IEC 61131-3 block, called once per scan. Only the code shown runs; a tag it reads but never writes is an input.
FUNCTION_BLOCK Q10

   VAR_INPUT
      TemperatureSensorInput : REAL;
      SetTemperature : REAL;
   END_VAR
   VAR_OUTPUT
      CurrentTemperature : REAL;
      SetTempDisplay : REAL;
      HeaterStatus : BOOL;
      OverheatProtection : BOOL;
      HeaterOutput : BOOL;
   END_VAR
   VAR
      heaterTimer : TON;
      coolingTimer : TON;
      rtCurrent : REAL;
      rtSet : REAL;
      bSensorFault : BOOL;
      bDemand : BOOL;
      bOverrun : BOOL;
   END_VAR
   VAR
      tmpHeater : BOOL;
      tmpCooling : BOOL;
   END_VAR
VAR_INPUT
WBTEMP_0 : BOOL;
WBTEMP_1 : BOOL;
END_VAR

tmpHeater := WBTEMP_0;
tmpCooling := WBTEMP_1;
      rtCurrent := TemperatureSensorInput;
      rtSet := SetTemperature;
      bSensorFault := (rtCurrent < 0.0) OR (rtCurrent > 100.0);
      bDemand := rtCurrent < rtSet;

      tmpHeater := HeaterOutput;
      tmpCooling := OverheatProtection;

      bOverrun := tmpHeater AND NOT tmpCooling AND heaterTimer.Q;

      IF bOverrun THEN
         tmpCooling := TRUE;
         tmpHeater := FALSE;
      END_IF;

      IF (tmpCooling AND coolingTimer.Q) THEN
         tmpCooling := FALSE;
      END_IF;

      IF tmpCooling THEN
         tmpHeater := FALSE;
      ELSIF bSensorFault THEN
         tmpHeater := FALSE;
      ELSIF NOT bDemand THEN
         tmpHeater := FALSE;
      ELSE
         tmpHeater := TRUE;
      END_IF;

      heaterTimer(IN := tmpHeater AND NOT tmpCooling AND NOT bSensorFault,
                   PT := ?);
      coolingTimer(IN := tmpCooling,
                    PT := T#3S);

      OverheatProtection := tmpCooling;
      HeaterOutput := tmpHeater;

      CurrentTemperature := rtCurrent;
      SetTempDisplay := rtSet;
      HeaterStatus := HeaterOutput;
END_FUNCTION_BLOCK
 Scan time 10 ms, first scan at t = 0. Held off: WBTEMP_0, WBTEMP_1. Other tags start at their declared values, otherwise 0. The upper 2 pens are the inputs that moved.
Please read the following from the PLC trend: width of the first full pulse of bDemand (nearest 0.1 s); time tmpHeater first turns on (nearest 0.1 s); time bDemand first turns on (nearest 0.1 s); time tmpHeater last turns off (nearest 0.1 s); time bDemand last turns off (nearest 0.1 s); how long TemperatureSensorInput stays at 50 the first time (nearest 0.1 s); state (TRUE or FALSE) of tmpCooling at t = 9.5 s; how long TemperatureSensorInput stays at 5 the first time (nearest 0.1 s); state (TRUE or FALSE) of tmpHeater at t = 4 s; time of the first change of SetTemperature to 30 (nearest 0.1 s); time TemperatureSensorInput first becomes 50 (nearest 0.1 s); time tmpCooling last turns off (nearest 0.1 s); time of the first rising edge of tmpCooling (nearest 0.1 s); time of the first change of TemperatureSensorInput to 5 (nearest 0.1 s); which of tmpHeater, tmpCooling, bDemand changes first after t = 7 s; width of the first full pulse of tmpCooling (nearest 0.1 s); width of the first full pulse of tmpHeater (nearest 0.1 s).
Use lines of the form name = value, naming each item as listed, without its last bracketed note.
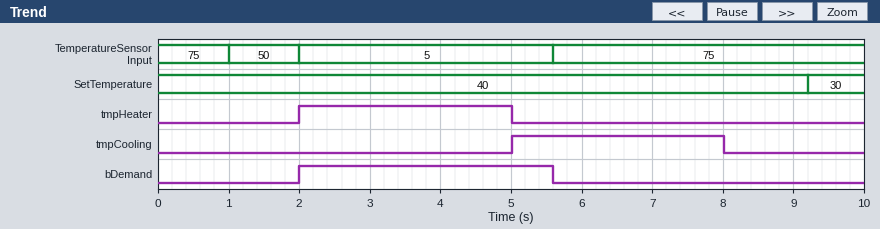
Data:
width of the first full pulse of bDemand = 3.6 s
time tmpHeater first turns on = 2.0 s
time bDemand first turns on = 2.0 s
time tmpHeater last turns off = 5.0 s
time bDemand last turns off = 5.6 s
how long TemperatureSensorInput stays at 50 the first time = 1.0 s
state (TRUE or FALSE) of tmpCooling at t = 9.5 s = FALSE
how long TemperatureSensorInput stays at 5 the first time = 3.6 s
state (TRUE or FALSE) of tmpHeater at t = 4 s = TRUE
time of the first change of SetTemperature to 30 = 9.2 s
time TemperatureSensorInput first becomes 50 = 1.0 s
time tmpCooling last turns off = 8.0 s
time of the first rising edge of tmpCooling = 5.0 s
time of the first change of TemperatureSensorInput to 5 = 2.0 s
which of tmpHeater, tmpCooling, bDemand changes first after t = 7 s = tmpCooling
width of the first full pulse of tmpCooling = 3.0 s
width of the first full pulse of tmpHeater = 3.0 s
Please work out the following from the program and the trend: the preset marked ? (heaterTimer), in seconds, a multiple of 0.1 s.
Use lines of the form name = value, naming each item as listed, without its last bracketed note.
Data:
the preset marked ? (heaterTimer), in seconds, a multiple of 0.1 s = 3.0 s
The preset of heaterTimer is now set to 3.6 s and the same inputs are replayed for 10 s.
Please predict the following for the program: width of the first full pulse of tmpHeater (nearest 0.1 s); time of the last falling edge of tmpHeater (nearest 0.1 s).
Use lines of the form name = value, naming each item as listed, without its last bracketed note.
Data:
width of the first full pulse of tmpHeater = 3.6 s
time of the last falling edge of tmpHeater = 5.6 s
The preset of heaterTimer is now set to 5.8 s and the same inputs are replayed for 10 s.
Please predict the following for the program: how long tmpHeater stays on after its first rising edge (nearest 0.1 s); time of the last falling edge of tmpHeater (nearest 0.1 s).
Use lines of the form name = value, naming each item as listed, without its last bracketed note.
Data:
how long tmpHeater stays on after its first rising edge = 3.6 s
time of the last falling edge of tmpHeater = 5.6 s
